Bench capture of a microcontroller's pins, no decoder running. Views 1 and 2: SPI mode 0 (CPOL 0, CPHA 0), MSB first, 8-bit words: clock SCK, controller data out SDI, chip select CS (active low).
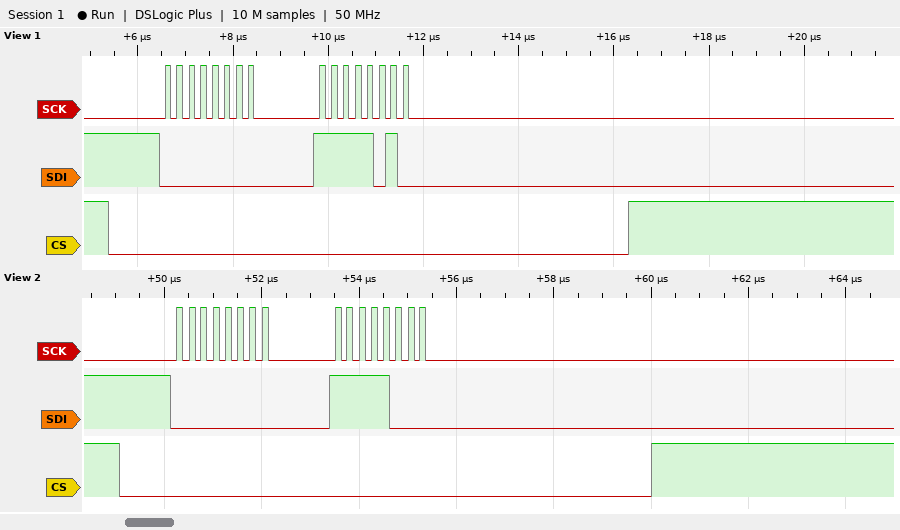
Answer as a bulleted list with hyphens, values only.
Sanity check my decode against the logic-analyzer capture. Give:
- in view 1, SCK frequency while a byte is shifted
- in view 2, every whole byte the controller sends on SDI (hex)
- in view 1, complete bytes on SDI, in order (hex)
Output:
- 4 MHz
- 0x00 0xF8
- 0x00 0xFA
